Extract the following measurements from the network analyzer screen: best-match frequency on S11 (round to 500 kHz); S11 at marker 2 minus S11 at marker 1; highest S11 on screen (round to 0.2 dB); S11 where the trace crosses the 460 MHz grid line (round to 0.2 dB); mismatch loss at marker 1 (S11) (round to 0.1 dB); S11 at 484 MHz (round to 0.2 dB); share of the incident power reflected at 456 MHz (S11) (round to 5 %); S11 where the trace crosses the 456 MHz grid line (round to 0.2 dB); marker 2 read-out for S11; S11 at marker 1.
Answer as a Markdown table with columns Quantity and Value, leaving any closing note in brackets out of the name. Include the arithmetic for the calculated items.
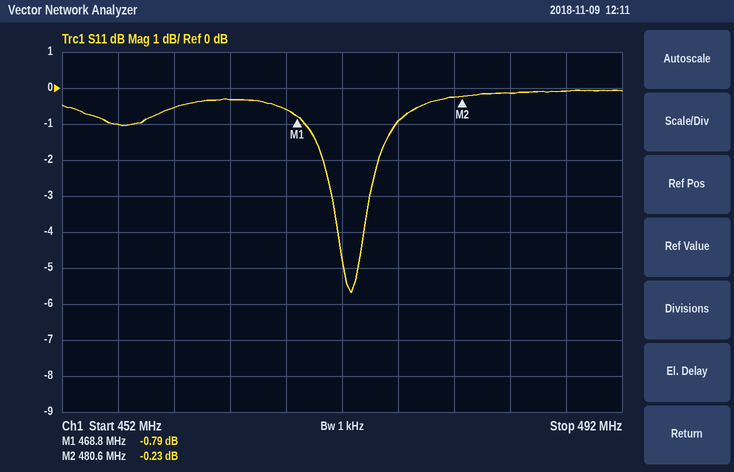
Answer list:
| Quantity | Value |
|---|---|
| best-match frequency on S11 | 472.5 MHz |
| S11 at marker 2 minus S11 at marker 1 | -0.23 − (-0.79) = 0.56 dB |
| highest S11 on screen | 0.0 dB |
| S11 where the trace crosses the 460 MHz grid line | -0.6 dB |
| mismatch loss at marker 1 (S11) | −10 log10(1 − 10^(-0.79/10)) ≈ 7.8 dB |
| S11 at 484 MHz | -0.2 dB |
| share of the incident power reflected at 456 MHz (S11) | 10^(-1/10) ≈ 79.4 %, so 80 % to the nearest 5 % |
| S11 where the trace crosses the 456 MHz grid line | -1.0 dB |
| marker 2 read-out for S11 | -0.23 dB |
| S11 at marker 1 | -0.79 dB |
